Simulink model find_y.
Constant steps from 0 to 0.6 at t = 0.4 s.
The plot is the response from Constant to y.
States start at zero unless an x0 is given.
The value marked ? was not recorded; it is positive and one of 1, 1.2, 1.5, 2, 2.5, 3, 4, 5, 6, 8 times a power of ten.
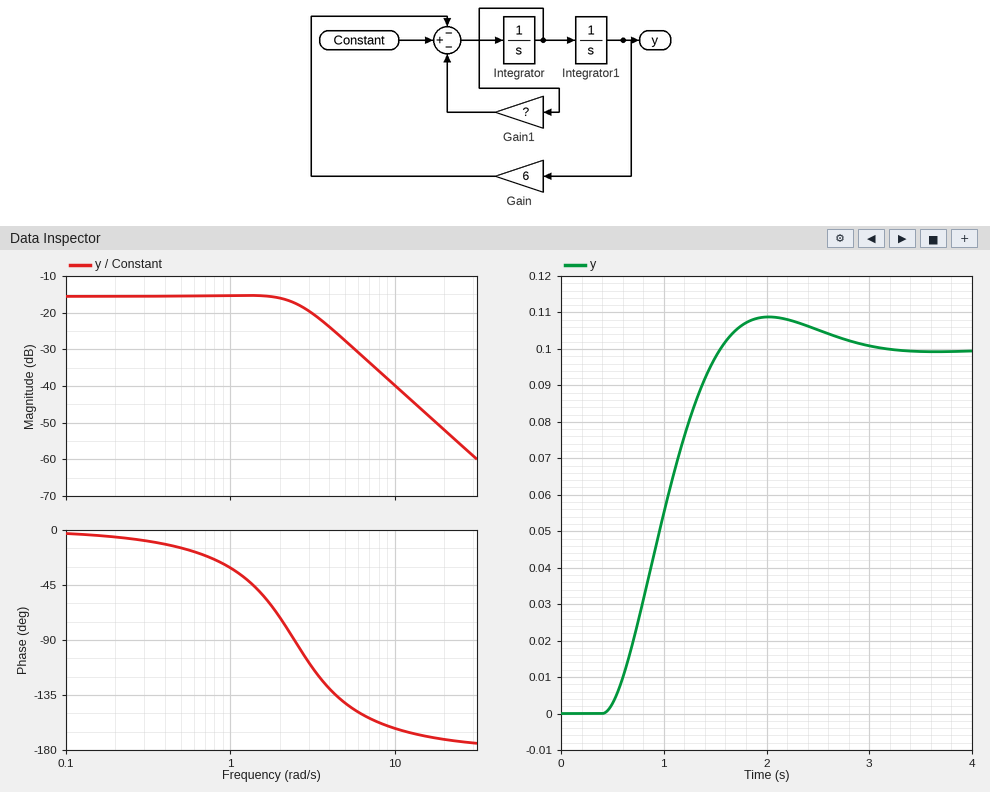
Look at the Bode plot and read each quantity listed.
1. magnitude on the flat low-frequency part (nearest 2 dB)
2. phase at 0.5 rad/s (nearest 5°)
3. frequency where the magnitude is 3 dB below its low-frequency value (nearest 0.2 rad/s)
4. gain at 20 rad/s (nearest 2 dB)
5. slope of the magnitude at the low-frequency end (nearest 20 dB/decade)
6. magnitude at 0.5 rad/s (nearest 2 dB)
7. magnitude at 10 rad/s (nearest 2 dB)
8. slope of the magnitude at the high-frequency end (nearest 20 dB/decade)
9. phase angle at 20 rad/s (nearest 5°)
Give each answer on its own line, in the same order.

-16 dB
-15°
2.8 rad/s
-52 dB
0 dB/decade
-16 dB
-40 dB
-40 dB/decade
-170°
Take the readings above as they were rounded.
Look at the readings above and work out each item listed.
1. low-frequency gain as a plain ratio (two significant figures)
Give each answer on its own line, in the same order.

0.16
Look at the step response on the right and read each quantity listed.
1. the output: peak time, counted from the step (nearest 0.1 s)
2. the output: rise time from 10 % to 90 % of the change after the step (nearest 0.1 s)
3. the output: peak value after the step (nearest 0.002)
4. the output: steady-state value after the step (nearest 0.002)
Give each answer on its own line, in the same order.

1.6 s
0.8 s
0.108
0.100
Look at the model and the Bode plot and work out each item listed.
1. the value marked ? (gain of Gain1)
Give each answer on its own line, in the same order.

3
